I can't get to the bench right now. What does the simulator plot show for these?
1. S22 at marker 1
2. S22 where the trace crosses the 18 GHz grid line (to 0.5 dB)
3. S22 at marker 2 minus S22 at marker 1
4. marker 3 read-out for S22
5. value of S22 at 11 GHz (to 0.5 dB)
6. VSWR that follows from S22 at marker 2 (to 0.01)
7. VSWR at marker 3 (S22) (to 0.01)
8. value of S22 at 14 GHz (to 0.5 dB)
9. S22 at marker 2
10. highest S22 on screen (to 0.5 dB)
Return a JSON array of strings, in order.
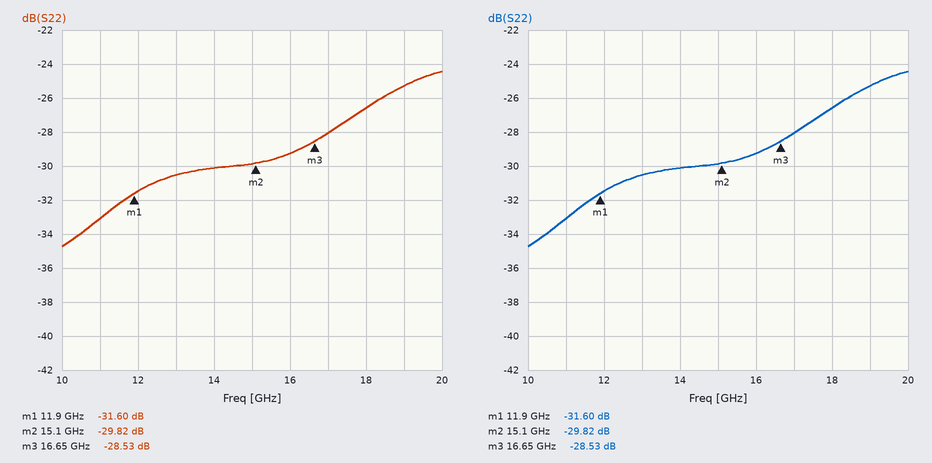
["-31.60 dB", "-26.5 dB", "1.78 dB", "-28.53 dB", "-33.0 dB", "1.07", "1.08", "-30.0 dB", "-29.82 dB", "-24.5 dB"]
